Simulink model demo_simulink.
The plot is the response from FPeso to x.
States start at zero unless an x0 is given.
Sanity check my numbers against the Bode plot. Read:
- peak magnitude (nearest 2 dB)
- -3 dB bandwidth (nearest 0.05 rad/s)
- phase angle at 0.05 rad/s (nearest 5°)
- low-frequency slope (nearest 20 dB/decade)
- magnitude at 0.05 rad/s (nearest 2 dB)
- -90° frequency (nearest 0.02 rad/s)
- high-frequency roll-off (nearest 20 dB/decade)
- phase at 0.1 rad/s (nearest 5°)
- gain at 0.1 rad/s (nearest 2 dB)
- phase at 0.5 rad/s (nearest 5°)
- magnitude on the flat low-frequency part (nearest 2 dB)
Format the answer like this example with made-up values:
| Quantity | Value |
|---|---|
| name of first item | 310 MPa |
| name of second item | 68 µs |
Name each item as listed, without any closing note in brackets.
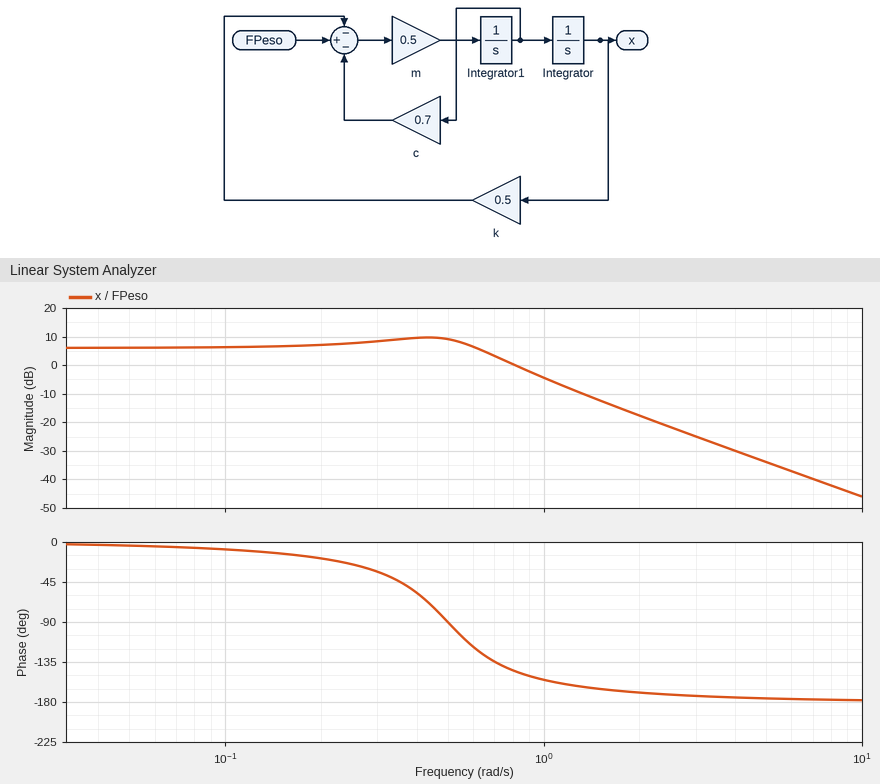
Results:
| Quantity | Value |
|---|---|
| peak magnitude | 10 dB |
| -3 dB bandwidth | 0.70 rad/s |
| phase angle at 0.05 rad/s | -5° |
| low-frequency slope | 0 dB/decade |
| magnitude at 0.05 rad/s | 6 dB |
| -90° frequency | 0.50 rad/s |
| high-frequency roll-off | -40 dB/decade |
| phase at 0.1 rad/s | -10° |
| gain at 0.1 rad/s | 6 dB |
| phase at 0.5 rad/s | -90° |
| magnitude on the flat low-frequency part | 6 dB |
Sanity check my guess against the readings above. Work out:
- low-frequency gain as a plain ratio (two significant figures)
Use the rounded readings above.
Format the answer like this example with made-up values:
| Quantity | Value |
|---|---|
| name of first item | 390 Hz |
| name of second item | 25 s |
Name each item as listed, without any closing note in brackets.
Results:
| Quantity | Value |
|---|---|
| low-frequency gain as a plain ratio | 2.0 |
